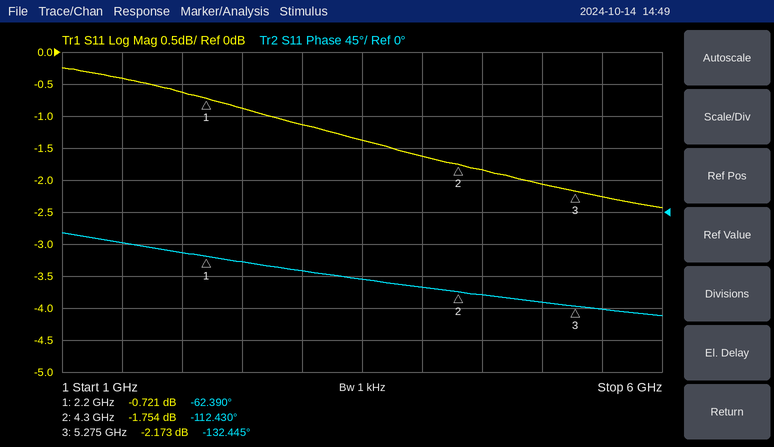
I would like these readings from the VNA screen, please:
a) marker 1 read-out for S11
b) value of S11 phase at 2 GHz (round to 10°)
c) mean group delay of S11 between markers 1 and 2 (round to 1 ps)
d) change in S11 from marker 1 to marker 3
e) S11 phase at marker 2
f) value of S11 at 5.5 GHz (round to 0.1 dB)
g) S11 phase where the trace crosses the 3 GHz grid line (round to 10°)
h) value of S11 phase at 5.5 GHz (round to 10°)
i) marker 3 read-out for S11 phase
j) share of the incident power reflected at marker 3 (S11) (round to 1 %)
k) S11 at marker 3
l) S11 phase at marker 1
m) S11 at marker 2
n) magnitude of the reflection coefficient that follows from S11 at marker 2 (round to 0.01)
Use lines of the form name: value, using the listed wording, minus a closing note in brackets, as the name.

marker 1 read-out for S11: -0.721 dB
value of S11 phase at 2 GHz: -60°
mean group delay of S11 between markers 1 and 2: 66 ps
change in S11 from marker 1 to marker 3: -1.452 dB
S11 phase at marker 2: -112.430°
value of S11 at 5.5 GHz: -2.3 dB
S11 phase where the trace crosses the 3 GHz grid line: -80°
value of S11 phase at 5.5 GHz: -140°
marker 3 read-out for S11 phase: -132.445°
share of the incident power reflected at marker 3 (S11): 61 %
S11 at marker 3: -2.173 dB
S11 phase at marker 1: -62.390°
S11 at marker 2: -1.754 dB
magnitude of the reflection coefficient that follows from S11 at marker 2: 0.82
